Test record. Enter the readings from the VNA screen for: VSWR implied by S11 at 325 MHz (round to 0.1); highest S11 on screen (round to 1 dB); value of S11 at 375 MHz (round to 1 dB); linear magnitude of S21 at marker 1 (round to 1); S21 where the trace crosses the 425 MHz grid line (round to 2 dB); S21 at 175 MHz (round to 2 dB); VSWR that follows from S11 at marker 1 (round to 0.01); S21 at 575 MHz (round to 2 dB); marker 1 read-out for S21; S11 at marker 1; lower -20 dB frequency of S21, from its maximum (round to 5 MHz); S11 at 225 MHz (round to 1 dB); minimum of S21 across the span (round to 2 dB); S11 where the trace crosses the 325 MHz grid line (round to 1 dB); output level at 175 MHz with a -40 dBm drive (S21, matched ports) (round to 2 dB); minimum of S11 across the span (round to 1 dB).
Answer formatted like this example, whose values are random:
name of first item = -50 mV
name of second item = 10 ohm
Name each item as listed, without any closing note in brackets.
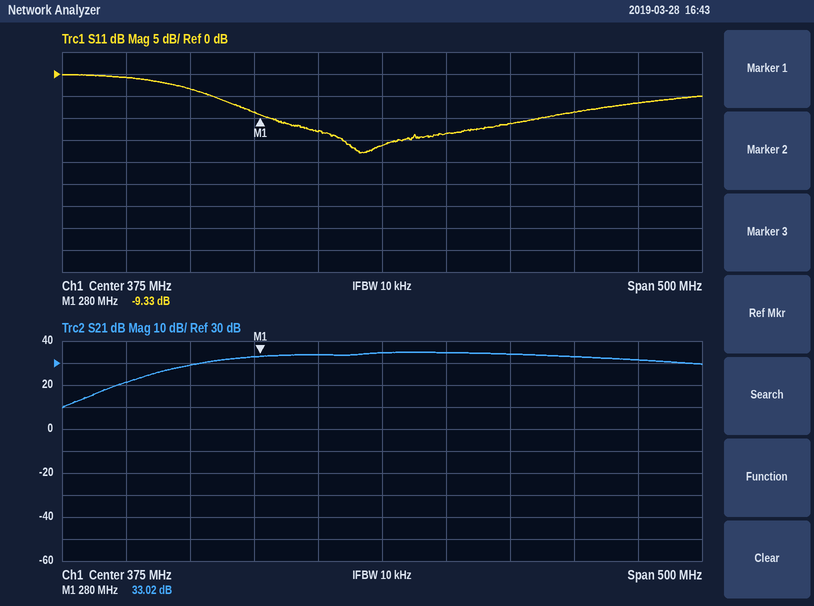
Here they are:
VSWR implied by S11 at 325 MHz = 1.6
highest S11 on screen = 0 dB
value of S11 at 375 MHz = -16 dB
linear magnitude of S21 at marker 1 = 45
S21 where the trace crosses the 425 MHz grid line = 34 dB
S21 at 175 MHz = 22 dB
VSWR that follows from S11 at marker 1 = 2.04
S21 at 575 MHz = 32 dB
marker 1 read-out for S21 = 33.02 dB
S11 at marker 1 = -9.33 dB
lower -20 dB frequency of S21, from its maximum = 145 MHz
S11 at 225 MHz = -3 dB
minimum of S21 across the span = 10 dB
S11 where the trace crosses the 325 MHz grid line = -13 dB
output level at 175 MHz with a -40 dBm drive (S21, matched ports) = -18 dBm
minimum of S11 across the span = -18 dB
